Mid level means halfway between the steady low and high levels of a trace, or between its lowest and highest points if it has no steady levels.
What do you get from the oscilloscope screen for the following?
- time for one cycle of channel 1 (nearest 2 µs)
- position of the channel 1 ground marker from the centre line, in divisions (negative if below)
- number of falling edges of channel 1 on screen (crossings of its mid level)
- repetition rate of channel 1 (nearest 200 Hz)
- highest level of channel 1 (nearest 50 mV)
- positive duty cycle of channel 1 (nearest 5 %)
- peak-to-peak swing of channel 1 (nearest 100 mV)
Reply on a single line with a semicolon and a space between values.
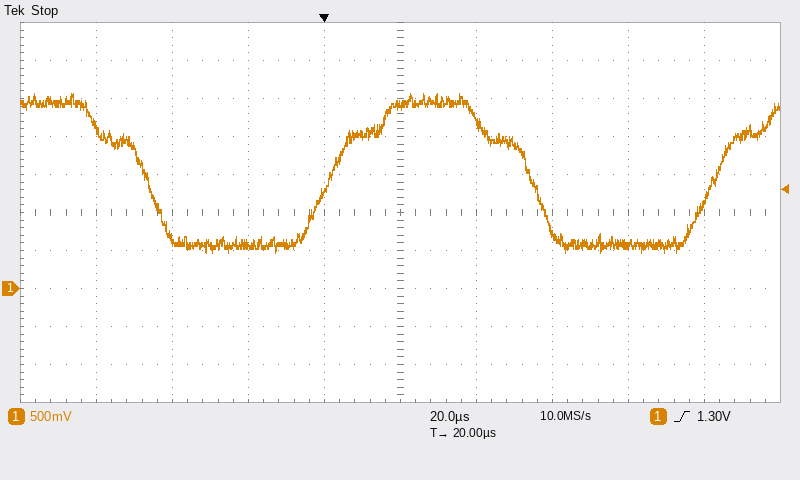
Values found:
102 µs; -2.0 div; 2; 9.8 kHz; 2.55 V; 50 %; 2.10 V
